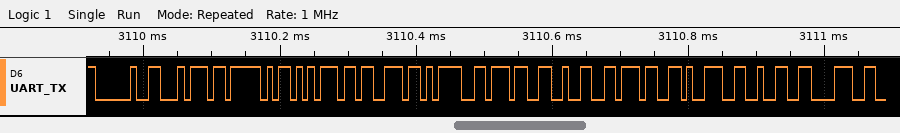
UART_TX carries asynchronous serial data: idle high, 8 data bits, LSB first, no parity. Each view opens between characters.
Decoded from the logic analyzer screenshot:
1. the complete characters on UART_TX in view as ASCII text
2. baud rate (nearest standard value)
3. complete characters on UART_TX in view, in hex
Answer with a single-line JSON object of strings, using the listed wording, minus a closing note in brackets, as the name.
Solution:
{"the complete characters on UART_TX in view as ASCII text": "\" t_us=727928\"", "baud rate": "115200 baud", "complete characters on UART_TX in view, in hex": "20, 74, 5F, 75, 73, 3D, 37, 32, 37, 39, 32, 38"}
